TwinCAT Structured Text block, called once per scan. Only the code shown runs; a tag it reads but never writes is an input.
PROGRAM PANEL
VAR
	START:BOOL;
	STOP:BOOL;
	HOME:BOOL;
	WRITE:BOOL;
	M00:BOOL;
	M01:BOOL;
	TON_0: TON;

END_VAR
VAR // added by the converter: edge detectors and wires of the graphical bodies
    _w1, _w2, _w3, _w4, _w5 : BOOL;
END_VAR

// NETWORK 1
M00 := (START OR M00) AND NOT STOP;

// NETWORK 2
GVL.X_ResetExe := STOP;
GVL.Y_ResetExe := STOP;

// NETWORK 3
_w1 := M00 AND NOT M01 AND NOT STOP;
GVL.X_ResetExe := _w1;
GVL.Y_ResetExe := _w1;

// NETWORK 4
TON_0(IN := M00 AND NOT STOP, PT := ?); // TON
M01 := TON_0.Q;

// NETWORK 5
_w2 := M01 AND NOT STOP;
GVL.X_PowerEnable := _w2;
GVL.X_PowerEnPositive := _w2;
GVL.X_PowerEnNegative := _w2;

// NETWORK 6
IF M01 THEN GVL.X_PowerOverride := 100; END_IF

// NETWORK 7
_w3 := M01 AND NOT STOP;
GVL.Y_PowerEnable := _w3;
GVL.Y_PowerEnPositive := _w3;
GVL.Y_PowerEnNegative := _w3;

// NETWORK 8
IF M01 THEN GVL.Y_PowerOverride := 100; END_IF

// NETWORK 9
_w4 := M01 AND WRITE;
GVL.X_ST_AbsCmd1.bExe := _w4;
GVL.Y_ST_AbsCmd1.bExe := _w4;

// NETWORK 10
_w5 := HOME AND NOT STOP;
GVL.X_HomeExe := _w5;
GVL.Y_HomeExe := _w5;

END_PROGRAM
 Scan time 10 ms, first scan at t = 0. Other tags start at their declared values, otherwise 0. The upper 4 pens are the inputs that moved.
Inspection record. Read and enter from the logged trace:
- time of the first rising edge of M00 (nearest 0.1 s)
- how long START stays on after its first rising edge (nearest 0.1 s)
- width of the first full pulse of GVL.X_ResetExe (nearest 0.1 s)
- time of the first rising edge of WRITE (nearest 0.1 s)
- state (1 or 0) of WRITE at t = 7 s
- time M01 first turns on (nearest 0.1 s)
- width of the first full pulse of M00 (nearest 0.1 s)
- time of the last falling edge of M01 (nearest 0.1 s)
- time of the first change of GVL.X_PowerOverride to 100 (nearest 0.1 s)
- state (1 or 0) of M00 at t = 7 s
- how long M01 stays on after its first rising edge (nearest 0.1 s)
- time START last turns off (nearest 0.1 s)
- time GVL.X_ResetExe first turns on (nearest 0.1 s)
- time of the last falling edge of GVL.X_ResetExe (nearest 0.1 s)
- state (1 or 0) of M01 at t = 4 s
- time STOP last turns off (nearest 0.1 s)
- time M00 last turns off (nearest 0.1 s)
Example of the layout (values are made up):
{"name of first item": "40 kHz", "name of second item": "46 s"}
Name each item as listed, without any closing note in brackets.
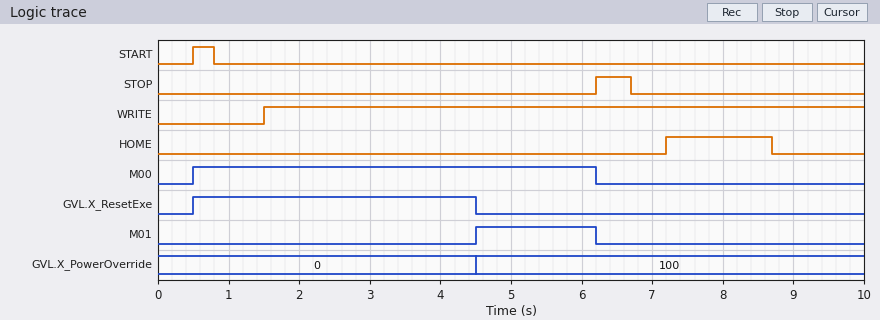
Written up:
{"time of the first rising edge of M00": "0.5 s", "how long START stays on after its first rising edge": "0.3 s", "width of the first full pulse of GVL.X_ResetExe": "4.0 s", "time of the first rising edge of WRITE": "1.5 s", "state (1 or 0) of WRITE at t = 7 s": "1", "time M01 first turns on": "4.5 s", "width of the first full pulse of M00": "5.7 s", "time of the last falling edge of M01": "6.2 s", "time of the first change of GVL.X_PowerOverride to 100": "4.5 s", "state (1 or 0) of M00 at t = 7 s": "0", "how long M01 stays on after its first rising edge": "1.7 s", "time START last turns off": "0.8 s", "time GVL.X_ResetExe first turns on": "0.5 s", "time of the last falling edge of GVL.X_ResetExe": "4.5 s", "state (1 or 0) of M01 at t = 4 s": "0", "time STOP last turns off": "6.7 s", "time M00 last turns off": "6.2 s"}
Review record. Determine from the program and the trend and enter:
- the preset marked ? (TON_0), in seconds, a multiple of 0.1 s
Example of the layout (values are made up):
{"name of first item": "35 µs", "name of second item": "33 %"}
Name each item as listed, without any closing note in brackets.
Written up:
{"the preset marked ? (TON_0), in seconds, a multiple of 0.1 s": "4.0 s"}
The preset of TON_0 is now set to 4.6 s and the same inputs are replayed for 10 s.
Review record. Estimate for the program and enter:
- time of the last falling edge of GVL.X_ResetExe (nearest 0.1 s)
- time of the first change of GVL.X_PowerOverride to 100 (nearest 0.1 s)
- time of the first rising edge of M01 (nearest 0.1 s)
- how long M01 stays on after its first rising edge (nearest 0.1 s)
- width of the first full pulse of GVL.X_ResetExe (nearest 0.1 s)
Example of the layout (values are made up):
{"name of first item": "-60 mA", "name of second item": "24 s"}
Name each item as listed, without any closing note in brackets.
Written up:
{"time of the last falling edge of GVL.X_ResetExe": "5.1 s", "time of the first change of GVL.X_PowerOverride to 100": "5.1 s", "time of the first rising edge of M01": "5.1 s", "how long M01 stays on after its first rising edge": "1.1 s", "width of the first full pulse of GVL.X_ResetExe": "4.6 s"}
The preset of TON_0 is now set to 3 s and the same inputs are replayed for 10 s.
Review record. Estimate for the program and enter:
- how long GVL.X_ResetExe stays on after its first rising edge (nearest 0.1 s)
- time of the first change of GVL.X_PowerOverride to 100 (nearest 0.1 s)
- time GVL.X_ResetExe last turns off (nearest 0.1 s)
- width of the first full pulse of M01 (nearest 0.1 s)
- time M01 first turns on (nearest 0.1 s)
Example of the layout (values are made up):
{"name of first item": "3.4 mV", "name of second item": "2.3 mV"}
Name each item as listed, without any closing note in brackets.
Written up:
{"how long GVL.X_ResetExe stays on after its first rising edge": "3.0 s", "time of the first change of GVL.X_PowerOverride to 100": "3.5 s", "time GVL.X_ResetExe last turns off": "3.5 s", "width of the first full pulse of M01": "2.7 s", "time M01 first turns on": "3.5 s"}
